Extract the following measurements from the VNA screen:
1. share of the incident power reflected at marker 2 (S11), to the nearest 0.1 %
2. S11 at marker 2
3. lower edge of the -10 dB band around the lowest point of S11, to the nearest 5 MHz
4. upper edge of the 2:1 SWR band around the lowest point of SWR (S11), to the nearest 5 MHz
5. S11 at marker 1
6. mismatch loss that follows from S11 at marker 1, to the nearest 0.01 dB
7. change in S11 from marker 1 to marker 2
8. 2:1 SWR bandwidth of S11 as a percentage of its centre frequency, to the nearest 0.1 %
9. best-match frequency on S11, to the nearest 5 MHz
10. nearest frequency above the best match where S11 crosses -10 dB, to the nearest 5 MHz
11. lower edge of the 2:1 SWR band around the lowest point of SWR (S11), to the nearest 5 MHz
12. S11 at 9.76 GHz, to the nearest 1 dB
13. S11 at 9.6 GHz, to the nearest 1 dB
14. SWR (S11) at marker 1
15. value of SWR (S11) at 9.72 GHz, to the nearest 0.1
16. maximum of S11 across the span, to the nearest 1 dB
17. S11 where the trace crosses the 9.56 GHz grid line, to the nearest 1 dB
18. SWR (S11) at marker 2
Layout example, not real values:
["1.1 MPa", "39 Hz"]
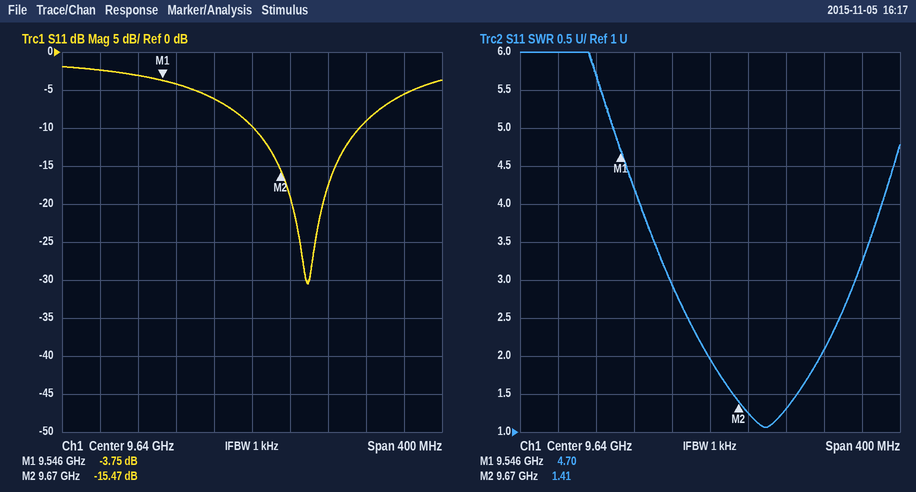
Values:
["2.8 %", "-15.47 dB", "9.640 GHz", "9.755 GHz", "-3.75 dB", "2.38 dB", "-11.72 dB", "1.2 %", "9.700 GHz", "9.755 GHz", "9.640 GHz", "-9 dB", "-6 dB", "4.70", "1.3", "-2 dB", "-4 dB", "1.41"]
